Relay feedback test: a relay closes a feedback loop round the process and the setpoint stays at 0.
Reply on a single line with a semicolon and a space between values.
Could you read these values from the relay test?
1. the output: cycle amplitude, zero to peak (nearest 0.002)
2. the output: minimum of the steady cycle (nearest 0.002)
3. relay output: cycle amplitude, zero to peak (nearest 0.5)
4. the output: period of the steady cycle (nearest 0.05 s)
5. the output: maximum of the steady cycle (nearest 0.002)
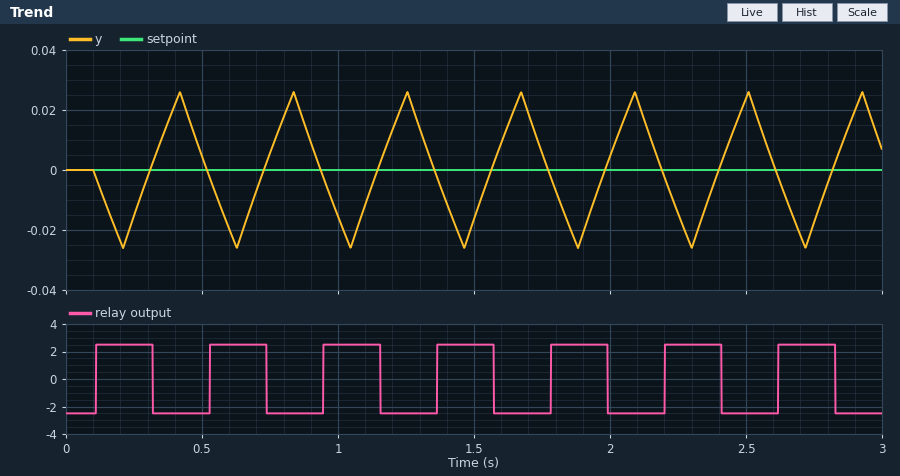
0.026; -0.026; 2.5; 0.40 s; 0.026
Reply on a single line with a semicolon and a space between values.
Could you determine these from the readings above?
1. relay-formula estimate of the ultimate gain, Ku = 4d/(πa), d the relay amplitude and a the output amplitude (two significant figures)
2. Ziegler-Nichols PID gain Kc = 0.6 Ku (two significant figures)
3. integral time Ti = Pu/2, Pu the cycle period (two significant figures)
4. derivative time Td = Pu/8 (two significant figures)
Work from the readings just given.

120; 72; 0.20 s; 0.050 s
